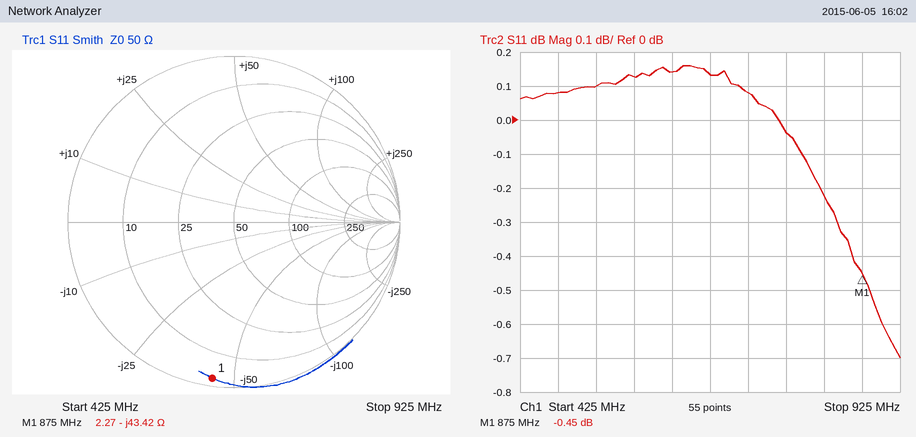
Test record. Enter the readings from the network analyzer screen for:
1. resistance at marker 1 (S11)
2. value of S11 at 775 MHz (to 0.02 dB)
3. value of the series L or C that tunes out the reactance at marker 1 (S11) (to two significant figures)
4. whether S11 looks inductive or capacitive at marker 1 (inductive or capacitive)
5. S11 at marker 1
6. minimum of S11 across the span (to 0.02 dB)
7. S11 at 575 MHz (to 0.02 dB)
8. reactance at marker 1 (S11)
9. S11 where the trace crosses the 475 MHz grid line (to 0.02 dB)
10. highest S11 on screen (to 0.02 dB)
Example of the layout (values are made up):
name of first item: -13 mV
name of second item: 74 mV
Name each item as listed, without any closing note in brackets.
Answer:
resistance at marker 1: 2.27 Ω
value of S11 at 775 MHz: -0.04 dB
value of the series L or C that tunes out the reactance at marker 1 (S11): 7.9 nH
whether S11 looks inductive or capacitive at marker 1: capacitive
S11 at marker 1: -0.45 dB
minimum of S11 across the span: -0.70 dB
S11 at 575 MHz: 0.12 dB
reactance at marker 1: -43.42 Ω
S11 where the trace crosses the 475 MHz grid line: 0.08 dB
highest S11 on screen: 0.16 dB
